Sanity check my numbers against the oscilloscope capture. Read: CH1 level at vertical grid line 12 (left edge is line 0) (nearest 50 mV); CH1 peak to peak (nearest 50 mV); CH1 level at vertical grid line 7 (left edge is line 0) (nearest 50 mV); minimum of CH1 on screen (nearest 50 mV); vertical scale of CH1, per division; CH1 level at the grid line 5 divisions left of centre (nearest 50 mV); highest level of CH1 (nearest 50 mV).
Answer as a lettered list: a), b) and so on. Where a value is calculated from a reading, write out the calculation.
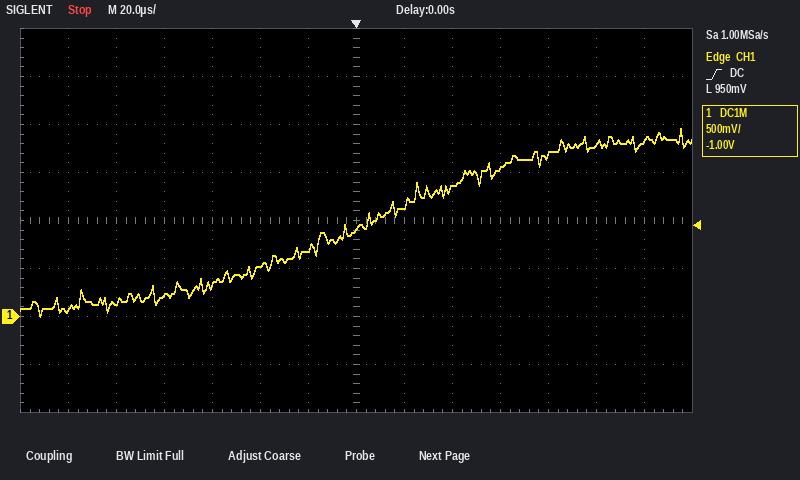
a) 1.80 V
b) 1.95 V − (0 mV) = 1.95 V
c) 900 mV
d) 0 mV
e) 500 mV
f) 150 mV
g) 1.95 V
